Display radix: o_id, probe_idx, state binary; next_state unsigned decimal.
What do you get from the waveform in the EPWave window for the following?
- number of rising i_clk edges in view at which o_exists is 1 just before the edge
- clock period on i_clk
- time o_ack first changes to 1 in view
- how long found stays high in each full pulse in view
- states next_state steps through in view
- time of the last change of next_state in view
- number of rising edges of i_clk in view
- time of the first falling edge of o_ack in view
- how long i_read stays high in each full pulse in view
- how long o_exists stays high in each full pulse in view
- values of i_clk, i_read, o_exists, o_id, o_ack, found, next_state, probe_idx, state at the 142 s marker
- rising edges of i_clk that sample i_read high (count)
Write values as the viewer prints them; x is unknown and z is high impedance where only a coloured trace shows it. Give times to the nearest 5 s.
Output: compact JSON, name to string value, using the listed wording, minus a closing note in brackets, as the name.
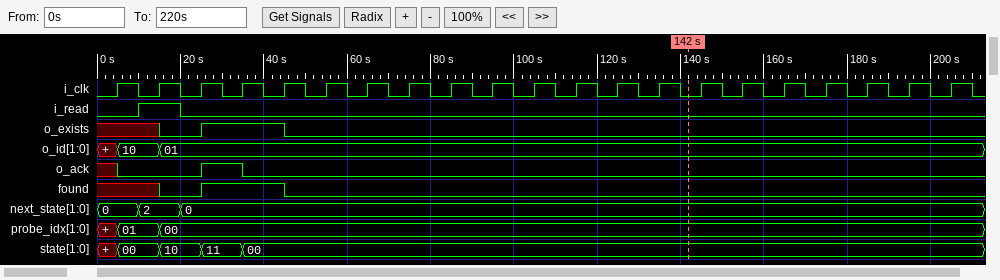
{"number of rising i_clk edges in view at which o_exists is 1 just before the edge": "2", "clock period on i_clk": "10 s", "time o_ack first changes to 1 in view": "25 s", "how long found stays high in each full pulse in view": "20 s", "states next_state steps through in view": "0, 2, 0", "time of the last change of next_state in view": "20 s", "number of rising edges of i_clk in view": "21", "time of the first falling edge of o_ack in view": "35 s", "how long i_read stays high in each full pulse in view": "10 s", "how long o_exists stays high in each full pulse in view": "20 s", "values of i_clk, i_read, o_exists, o_id, o_ack, found, next_state, probe_idx, state at the 142 s marker": "i_clk=0, i_read=0, o_exists=0, o_id=01, o_ack=0, found=0, next_state=0, probe_idx=00, state=00", "rising edges of i_clk that sample i_read high": "1"}
